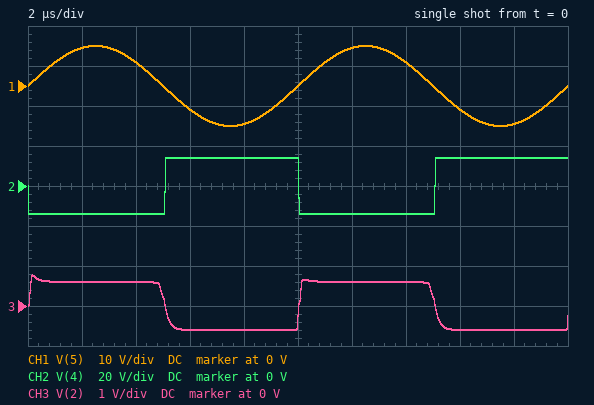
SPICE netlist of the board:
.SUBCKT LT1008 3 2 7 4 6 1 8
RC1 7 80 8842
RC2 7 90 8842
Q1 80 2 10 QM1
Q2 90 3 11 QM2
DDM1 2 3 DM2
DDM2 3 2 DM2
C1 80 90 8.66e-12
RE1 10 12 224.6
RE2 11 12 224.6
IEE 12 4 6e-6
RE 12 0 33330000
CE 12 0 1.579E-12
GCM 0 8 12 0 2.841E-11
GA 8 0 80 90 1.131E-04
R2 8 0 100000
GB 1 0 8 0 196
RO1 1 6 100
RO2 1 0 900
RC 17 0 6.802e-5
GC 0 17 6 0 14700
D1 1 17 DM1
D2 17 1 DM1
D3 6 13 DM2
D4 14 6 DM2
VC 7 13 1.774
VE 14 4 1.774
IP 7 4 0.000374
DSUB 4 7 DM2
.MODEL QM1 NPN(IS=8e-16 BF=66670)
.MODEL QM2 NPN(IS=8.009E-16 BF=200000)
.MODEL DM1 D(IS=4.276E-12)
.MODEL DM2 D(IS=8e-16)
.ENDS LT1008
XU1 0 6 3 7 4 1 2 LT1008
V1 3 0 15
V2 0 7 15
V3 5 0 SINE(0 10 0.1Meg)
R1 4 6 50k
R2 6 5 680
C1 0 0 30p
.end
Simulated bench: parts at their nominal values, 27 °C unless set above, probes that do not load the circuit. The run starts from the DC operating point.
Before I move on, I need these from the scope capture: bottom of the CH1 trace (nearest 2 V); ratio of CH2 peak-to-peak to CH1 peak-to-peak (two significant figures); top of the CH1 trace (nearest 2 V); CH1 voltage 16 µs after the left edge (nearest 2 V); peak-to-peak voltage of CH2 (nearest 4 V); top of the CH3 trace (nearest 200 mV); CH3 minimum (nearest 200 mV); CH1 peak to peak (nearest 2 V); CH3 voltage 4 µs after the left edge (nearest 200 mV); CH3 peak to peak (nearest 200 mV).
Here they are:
-10 V
1.4
10 V
-6 V
28 V
800 mV
-600 mV
20 V
600 mV
1.4 V
